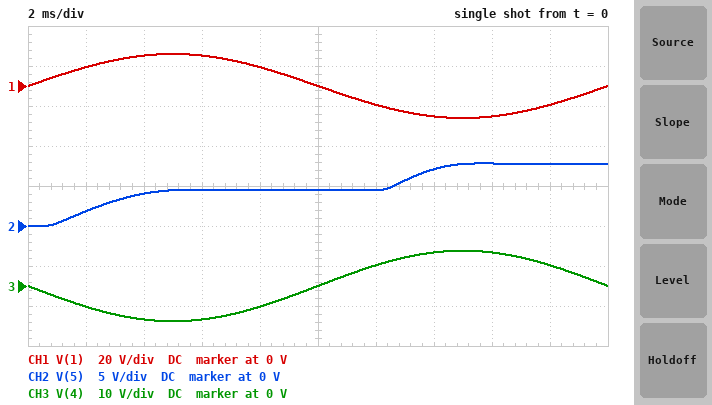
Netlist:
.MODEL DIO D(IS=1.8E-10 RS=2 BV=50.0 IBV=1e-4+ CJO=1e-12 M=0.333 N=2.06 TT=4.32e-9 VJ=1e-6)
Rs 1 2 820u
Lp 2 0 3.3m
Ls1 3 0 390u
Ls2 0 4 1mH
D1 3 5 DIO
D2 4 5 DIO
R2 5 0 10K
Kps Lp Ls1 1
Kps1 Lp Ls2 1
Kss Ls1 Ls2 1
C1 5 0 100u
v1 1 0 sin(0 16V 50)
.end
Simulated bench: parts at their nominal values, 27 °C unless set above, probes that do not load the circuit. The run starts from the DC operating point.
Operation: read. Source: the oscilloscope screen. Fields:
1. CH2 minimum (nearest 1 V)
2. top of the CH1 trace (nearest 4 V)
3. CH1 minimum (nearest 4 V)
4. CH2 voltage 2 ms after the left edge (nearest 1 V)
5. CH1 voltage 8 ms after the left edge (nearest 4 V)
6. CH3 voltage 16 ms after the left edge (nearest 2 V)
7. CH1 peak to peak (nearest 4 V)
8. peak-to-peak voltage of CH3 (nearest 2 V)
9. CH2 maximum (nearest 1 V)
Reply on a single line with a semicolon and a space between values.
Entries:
0 V; 16 V; -16 V; 2 V; 8 V; 8 V; 32 V; 18 V; 8 V
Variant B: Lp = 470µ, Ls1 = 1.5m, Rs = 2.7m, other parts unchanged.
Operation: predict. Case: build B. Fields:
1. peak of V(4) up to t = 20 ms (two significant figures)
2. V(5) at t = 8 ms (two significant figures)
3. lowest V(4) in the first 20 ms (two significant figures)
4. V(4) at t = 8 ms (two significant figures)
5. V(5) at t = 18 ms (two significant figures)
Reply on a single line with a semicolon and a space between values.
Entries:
24 V; 27 V; -23 V; -13 V; 22 V
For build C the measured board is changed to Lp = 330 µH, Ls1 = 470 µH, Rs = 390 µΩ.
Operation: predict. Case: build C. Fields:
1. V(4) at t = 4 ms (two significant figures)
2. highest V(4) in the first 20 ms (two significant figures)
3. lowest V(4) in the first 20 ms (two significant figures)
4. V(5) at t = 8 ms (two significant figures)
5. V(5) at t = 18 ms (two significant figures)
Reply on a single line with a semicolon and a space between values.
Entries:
-26 V; 28 V; -28 V; 18 V; 27 V
